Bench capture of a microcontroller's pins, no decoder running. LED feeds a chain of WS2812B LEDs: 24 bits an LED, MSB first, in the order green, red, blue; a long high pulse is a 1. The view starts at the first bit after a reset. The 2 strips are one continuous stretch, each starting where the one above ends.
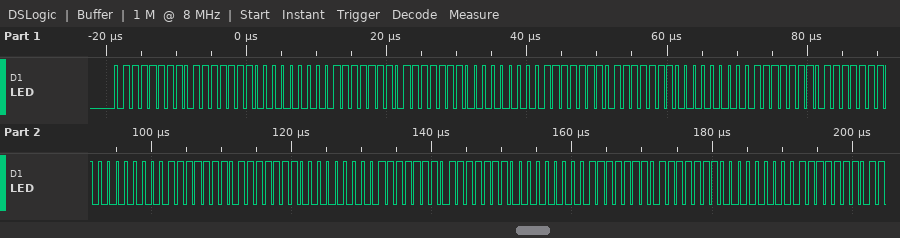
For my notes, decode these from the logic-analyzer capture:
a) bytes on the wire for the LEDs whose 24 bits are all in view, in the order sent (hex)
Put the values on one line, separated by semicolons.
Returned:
7F 7F 00 7F 7F 00 7F 7F 00 7F 7F 00 7F 7F 00 7F 7F 00 7F 7F 00
